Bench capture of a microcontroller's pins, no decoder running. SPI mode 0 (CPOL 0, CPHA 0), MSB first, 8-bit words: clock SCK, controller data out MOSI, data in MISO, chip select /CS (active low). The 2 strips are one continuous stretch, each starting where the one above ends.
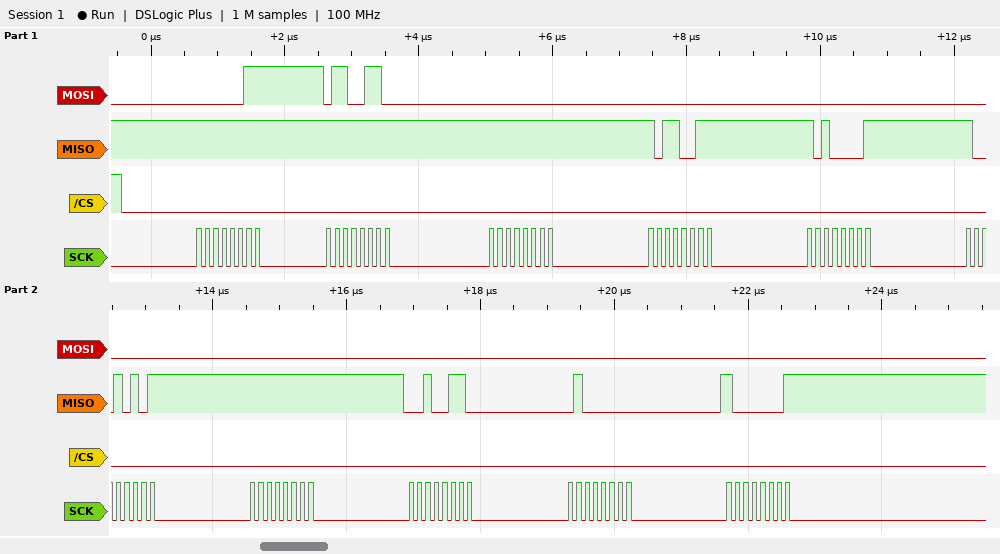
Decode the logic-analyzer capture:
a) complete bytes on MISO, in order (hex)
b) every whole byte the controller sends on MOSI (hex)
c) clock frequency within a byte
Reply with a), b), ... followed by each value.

a) FF FF FF B3 A1 95 FF 26 40 81
b) 03 66 00 00 00 00 00 00 00 00
c) 8 MHz
